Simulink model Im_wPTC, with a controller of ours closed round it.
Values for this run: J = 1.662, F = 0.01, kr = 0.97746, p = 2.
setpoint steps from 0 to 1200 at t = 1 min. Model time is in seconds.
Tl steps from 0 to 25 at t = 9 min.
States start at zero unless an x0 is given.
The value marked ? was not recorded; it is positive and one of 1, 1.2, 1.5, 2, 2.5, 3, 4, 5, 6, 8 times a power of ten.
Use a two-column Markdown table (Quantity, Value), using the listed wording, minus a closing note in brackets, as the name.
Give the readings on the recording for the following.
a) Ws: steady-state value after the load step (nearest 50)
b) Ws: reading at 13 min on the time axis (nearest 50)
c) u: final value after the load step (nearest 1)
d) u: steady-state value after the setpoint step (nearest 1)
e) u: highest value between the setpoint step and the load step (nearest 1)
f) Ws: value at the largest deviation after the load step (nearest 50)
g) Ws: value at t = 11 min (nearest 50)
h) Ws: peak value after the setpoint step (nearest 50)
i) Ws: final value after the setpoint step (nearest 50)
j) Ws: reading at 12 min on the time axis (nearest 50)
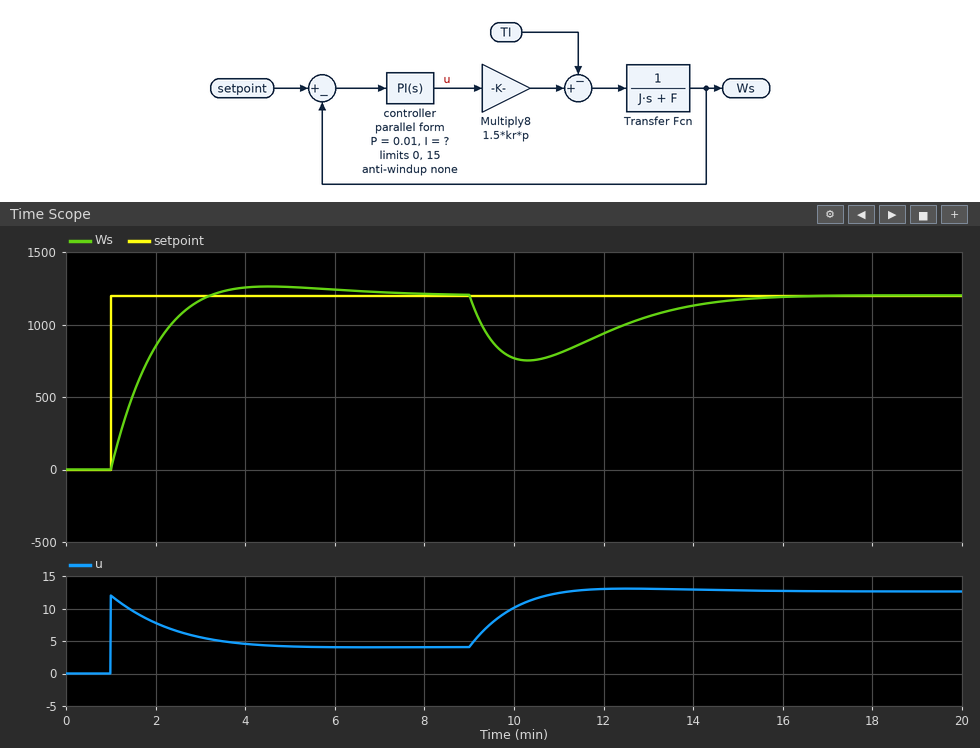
| Quantity | Value |
|---|---|
| Ws: steady-state value after the load step | 1200 |
| Ws: reading at 13 min on the time axis | 1050 |
| u: final value after the load step | 13 |
| u: steady-state value after the setpoint step | 4 |
| u: highest value between the setpoint step and the load step | 12 |
| Ws: value at the largest deviation after the load step | 750 |
| Ws: value at t = 11 min | 800 |
| Ws: peak value after the setpoint step | 1250 |
| Ws: final value after the setpoint step | 1200 |
| Ws: reading at 12 min on the time axis | 950 |
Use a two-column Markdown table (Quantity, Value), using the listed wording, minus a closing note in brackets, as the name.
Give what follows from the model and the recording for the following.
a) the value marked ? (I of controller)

| Quantity | Value |
|---|---|
| the value marked ? | 0.0001 |
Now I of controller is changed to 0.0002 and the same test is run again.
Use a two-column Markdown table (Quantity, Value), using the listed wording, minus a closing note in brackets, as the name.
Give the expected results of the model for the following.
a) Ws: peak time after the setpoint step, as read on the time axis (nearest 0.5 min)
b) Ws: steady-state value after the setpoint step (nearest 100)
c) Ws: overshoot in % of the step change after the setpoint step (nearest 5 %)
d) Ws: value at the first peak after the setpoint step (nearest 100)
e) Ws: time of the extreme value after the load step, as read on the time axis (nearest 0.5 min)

| Quantity | Value |
|---|---|
| Ws: peak time after the setpoint step, as read on the time axis | 3.5 min |
| Ws: steady-state value after the setpoint step | 1200 |
| Ws: overshoot in % of the step change after the setpoint step | 15 % |
| Ws: value at the first peak after the setpoint step | 1400 |
| Ws: time of the extreme value after the load step, as read on the time axis | 10.0 min |
